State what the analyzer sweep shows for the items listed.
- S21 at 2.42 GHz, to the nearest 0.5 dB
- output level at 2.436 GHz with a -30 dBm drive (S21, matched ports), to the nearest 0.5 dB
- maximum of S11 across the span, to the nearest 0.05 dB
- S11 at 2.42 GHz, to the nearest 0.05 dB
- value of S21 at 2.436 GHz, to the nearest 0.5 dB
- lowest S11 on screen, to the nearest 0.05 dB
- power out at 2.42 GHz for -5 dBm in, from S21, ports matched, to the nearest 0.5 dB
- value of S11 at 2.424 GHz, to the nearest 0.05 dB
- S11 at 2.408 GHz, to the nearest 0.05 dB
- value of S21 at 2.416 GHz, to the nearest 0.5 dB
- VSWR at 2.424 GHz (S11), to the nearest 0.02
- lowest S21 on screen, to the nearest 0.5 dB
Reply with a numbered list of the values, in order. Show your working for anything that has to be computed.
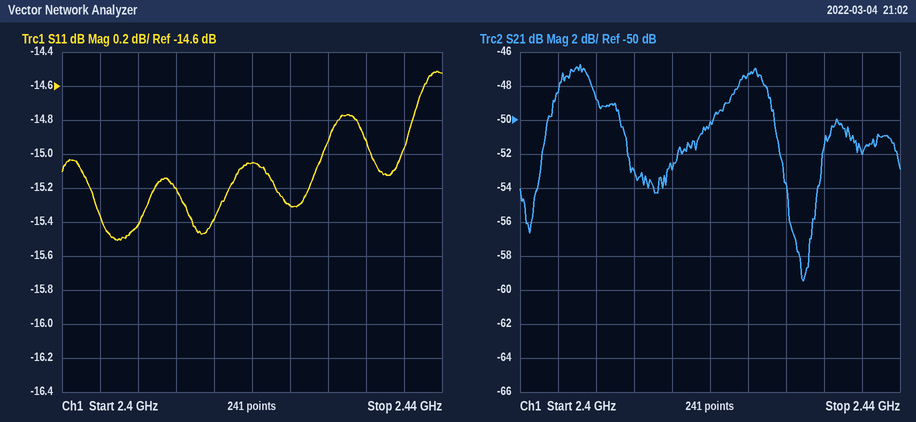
1. -50.0 dB
2. -30 dBm + (-52.0 dB) = -82.0 dBm
3. -14.50 dB
4. -15.05 dB
5. -52.0 dB
6. -15.50 dB
7. -5 dBm + (-50.0 dB) = -55.0 dBm
8. -15.30 dB
9. -15.40 dB
10. -53.0 dB
11. |Γ| = 10^(-15.3/20) = 0.1718; VSWR = (1 + 0.1718)/(1 − 0.1718) ≈ 1.41, so 1.42 to the nearest 0.02
12. -59.5 dB
